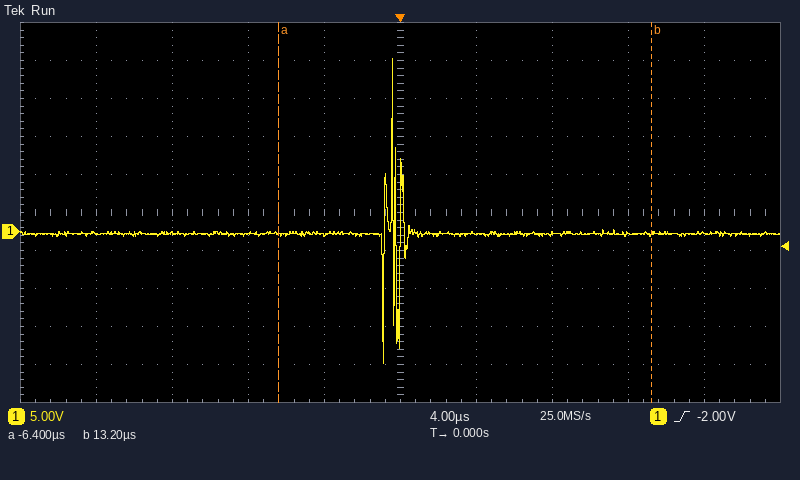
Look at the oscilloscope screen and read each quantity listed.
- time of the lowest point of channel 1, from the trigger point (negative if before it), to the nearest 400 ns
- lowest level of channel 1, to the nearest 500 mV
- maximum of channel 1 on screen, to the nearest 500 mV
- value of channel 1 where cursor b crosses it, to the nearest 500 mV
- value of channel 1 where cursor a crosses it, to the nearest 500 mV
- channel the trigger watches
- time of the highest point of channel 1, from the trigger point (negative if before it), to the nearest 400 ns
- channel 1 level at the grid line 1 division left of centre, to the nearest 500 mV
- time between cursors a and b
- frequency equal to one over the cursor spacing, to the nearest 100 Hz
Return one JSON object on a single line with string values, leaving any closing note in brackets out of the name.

{"time of the lowest point of channel 1, from the trigger point (negative if before it), to the nearest 400 ns": "-800 ns", "lowest level of channel 1, to the nearest 500 mV": "-17.5 V", "maximum of channel 1 on screen, to the nearest 500 mV": "23.0 V", "value of channel 1 where cursor b crosses it, to the nearest 500 mV": "-500 mV", "value of channel 1 where cursor a crosses it, to the nearest 500 mV": "-500 mV", "channel the trigger watches": "channel 1", "time of the highest point of channel 1, from the trigger point (negative if before it), to the nearest 400 ns": "-400 ns", "channel 1 level at the grid line 1 division left of centre, to the nearest 500 mV": "-500 mV", "time between cursors a and b": "19.6 µs", "frequency equal to one over the cursor spacing, to the nearest 100 Hz": "51.0 kHz"}
